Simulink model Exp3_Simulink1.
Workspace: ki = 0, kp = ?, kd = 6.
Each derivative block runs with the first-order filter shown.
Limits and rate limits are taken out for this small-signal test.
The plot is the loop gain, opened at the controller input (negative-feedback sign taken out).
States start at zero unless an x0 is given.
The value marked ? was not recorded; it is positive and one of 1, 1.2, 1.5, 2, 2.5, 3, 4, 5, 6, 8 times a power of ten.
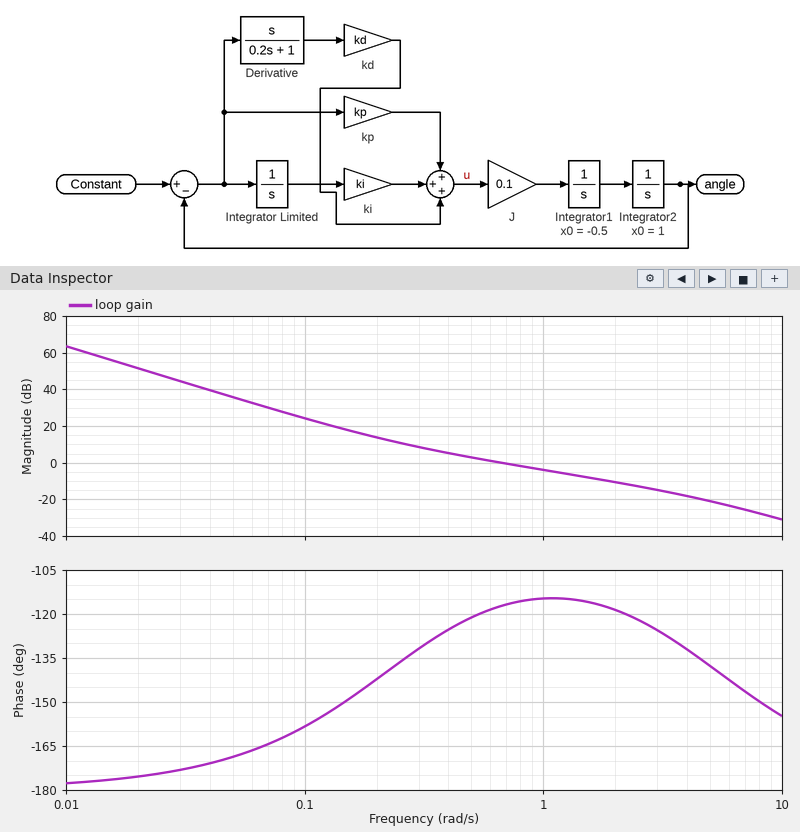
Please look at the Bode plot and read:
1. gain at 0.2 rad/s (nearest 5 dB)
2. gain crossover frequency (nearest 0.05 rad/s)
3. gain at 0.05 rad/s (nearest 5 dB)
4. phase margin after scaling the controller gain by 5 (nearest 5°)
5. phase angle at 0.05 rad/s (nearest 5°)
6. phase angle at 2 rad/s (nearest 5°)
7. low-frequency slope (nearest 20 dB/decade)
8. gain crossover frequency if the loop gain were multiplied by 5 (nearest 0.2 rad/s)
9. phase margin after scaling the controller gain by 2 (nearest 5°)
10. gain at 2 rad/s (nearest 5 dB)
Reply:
15 dB
0.65 rad/s
35 dB
55°
-170°
-120°
-40 dB/decade
2.8 rad/s
65°
-10 dB
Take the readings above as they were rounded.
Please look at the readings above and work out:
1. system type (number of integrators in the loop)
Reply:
2
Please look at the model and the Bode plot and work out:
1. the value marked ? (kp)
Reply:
1.5
